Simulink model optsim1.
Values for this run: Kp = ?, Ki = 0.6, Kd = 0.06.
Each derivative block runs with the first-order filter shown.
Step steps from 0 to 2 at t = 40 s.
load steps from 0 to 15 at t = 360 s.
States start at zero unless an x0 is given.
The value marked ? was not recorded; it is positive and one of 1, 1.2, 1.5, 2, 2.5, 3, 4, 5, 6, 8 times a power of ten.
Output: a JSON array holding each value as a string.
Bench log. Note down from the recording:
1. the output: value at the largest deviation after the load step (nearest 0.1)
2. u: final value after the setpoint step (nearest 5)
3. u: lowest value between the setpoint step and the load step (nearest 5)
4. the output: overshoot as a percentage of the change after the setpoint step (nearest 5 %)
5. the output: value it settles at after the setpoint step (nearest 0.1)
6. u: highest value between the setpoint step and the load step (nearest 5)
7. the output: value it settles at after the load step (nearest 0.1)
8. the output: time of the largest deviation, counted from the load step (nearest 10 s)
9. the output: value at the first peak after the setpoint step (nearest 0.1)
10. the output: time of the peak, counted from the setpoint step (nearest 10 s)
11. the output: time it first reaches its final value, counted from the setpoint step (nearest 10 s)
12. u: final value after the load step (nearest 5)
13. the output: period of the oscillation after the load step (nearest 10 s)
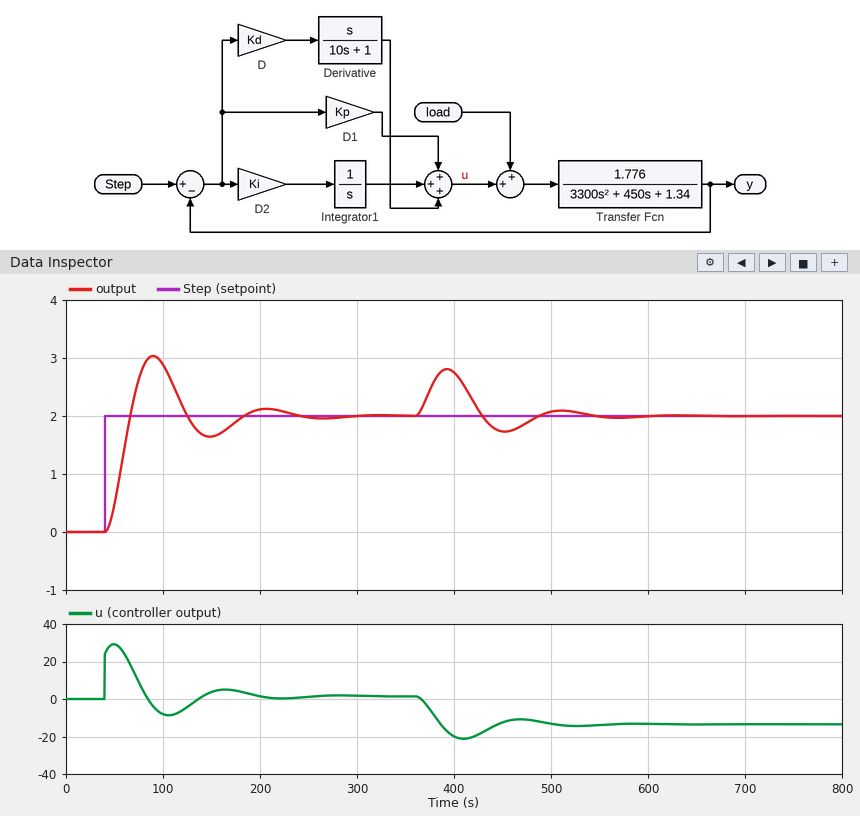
["2.8", "0", "-10", "50 %", "2.0", "30", "2.0", "30 s", "3.0", "50 s", "30 s", "-15", "120 s"]
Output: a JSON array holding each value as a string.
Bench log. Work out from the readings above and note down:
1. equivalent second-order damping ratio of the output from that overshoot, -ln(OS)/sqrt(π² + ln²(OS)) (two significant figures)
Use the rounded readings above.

["0.22"]
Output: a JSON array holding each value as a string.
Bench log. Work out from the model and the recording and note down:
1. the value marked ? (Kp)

["12"]
